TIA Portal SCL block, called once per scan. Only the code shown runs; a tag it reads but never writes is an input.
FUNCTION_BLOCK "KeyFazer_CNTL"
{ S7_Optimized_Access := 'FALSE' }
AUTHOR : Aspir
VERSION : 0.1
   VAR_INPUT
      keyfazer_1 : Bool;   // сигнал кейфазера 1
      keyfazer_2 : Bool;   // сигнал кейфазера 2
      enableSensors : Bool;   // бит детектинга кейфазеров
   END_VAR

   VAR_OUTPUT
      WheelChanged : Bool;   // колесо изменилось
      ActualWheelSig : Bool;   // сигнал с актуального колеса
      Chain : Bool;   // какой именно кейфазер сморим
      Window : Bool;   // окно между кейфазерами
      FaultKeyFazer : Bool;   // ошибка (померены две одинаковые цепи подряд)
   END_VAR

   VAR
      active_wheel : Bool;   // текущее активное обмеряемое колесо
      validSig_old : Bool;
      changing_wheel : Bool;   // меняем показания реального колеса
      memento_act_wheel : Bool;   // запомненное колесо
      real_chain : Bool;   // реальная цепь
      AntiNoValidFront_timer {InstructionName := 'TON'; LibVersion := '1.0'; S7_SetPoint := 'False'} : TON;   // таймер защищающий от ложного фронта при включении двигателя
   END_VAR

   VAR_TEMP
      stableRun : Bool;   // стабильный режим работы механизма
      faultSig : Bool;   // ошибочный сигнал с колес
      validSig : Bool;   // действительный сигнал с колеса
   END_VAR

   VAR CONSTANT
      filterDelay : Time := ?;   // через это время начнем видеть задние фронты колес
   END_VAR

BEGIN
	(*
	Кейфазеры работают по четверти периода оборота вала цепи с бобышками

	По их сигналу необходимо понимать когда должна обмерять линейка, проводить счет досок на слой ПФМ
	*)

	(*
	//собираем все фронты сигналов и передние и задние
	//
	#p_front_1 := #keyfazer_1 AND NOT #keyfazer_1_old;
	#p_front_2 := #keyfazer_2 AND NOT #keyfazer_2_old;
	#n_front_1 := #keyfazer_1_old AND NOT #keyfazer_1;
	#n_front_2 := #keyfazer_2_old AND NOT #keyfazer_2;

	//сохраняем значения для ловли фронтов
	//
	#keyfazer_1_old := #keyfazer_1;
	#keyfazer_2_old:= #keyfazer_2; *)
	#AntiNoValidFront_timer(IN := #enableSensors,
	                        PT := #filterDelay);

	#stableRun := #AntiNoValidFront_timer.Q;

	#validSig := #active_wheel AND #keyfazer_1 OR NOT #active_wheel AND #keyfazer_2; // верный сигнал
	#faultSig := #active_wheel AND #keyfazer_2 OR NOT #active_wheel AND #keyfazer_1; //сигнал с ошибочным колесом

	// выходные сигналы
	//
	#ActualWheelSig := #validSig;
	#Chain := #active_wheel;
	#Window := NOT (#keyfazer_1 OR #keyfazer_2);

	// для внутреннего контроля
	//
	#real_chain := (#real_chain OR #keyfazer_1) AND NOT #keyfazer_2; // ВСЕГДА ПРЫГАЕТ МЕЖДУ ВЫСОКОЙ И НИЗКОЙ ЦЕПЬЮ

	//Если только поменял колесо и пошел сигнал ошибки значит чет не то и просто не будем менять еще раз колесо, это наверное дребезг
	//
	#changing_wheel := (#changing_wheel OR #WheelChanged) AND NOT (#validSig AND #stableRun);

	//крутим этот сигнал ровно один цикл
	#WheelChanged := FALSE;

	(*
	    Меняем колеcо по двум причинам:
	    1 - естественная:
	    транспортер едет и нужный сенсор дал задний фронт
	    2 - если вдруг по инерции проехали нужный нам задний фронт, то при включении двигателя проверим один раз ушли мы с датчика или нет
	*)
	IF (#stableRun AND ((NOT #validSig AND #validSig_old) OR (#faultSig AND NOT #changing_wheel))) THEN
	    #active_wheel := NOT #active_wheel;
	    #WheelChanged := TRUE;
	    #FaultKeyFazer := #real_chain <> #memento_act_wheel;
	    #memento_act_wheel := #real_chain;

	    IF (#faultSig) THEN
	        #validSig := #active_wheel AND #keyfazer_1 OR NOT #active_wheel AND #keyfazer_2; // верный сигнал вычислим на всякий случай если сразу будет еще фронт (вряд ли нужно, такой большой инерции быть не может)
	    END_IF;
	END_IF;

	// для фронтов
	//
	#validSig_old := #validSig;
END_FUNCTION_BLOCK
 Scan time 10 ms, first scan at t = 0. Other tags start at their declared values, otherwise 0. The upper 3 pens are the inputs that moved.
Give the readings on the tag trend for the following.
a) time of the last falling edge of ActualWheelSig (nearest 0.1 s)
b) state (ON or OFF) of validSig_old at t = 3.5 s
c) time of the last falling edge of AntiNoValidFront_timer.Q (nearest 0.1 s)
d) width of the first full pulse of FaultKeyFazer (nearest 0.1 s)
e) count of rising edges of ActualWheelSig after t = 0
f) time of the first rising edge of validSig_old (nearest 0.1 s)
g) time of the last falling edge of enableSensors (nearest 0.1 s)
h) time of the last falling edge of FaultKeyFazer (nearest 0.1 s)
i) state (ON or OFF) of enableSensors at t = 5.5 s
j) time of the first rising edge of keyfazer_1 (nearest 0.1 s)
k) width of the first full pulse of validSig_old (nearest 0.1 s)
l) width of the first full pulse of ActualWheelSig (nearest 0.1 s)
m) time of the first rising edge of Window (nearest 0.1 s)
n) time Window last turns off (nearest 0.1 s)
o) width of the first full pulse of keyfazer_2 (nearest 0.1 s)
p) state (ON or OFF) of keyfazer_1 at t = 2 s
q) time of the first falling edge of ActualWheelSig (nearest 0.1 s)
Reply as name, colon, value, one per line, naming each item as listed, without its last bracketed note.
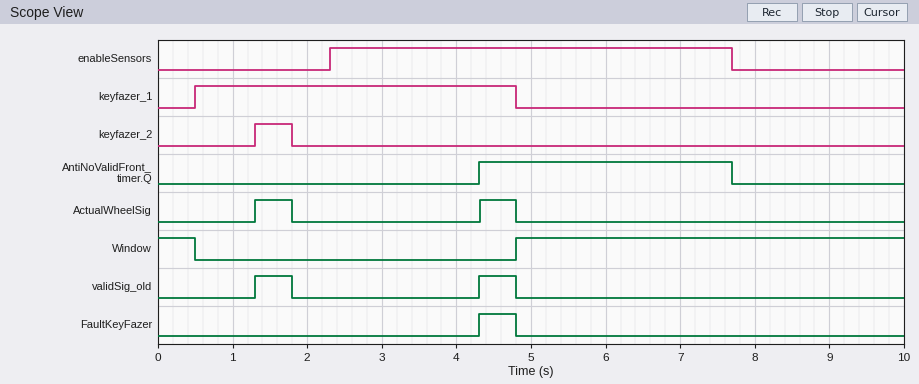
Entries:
time of the last falling edge of ActualWheelSig: 4.8 s
state (ON or OFF) of validSig_old at t = 3.5 s: OFF
time of the last falling edge of AntiNoValidFront_timer.Q: 7.7 s
width of the first full pulse of FaultKeyFazer: 0.5 s
count of rising edges of ActualWheelSig after t = 0: 2
time of the first rising edge of validSig_old: 1.3 s
time of the last falling edge of enableSensors: 7.7 s
time of the last falling edge of FaultKeyFazer: 4.8 s
state (ON or OFF) of enableSensors at t = 5.5 s: ON
time of the first rising edge of keyfazer_1: 0.5 s
width of the first full pulse of validSig_old: 0.5 s
width of the first full pulse of ActualWheelSig: 0.5 s
time of the first rising edge of Window: 4.8 s
time Window last turns off: 0.5 s
width of the first full pulse of keyfazer_2: 0.5 s
state (ON or OFF) of keyfazer_1 at t = 2 s: ON
time of the first falling edge of ActualWheelSig: 1.8 s
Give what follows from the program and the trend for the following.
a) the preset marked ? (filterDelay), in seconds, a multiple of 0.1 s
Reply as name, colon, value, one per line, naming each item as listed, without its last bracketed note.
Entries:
the preset marked ? (filterDelay), in seconds, a multiple of 0.1 s: 2.0 s
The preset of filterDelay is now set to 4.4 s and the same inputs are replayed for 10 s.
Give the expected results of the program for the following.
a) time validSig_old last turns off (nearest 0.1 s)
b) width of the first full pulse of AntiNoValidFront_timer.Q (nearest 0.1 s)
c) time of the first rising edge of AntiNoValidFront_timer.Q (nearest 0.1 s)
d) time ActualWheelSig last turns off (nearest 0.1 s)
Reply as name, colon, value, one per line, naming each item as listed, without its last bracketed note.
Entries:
time validSig_old last turns off: 1.8 s
width of the first full pulse of AntiNoValidFront_timer.Q: 1.0 s
time of the first rising edge of AntiNoValidFront_timer.Q: 6.7 s
time ActualWheelSig last turns off: 1.8 s
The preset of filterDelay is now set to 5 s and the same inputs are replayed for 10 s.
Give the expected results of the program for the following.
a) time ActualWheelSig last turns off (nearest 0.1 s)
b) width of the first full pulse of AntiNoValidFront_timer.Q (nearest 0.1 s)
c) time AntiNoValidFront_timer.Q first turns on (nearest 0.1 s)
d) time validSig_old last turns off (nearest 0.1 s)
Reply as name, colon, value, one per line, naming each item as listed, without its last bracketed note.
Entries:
time ActualWheelSig last turns off: 1.8 s
width of the first full pulse of AntiNoValidFront_timer.Q: 0.4 s
time AntiNoValidFront_timer.Q first turns on: 7.3 s
time validSig_old last turns off: 1.8 s
